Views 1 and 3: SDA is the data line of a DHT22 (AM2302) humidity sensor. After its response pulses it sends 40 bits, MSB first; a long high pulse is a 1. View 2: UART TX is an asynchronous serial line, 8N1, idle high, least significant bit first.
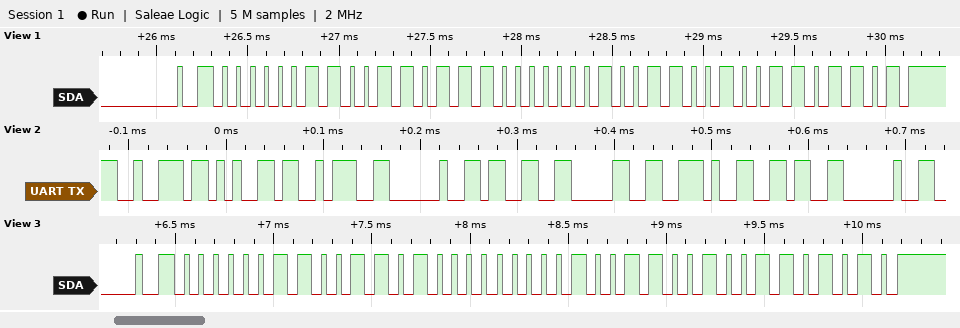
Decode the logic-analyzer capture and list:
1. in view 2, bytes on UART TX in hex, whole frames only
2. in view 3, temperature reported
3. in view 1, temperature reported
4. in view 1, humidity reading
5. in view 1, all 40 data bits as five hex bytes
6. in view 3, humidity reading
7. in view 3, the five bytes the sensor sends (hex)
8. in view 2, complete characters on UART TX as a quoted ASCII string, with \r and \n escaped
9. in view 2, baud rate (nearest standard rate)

72 65 3A 20 33 30 2E 36 20
30.6 °C
30.6 °C
82.3 %
03 37 01 32 6D
82.0 %
03 34 01 32 6A
"re: 30.6 "
115200 baud
